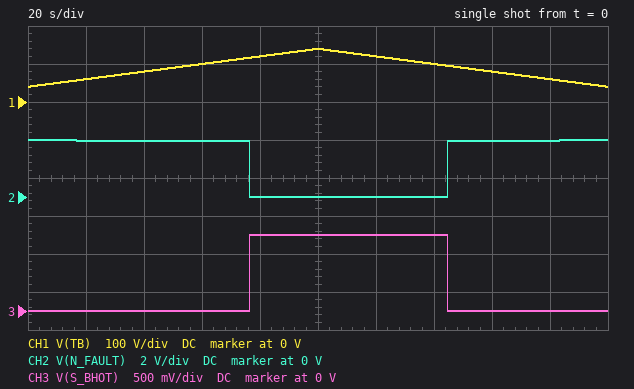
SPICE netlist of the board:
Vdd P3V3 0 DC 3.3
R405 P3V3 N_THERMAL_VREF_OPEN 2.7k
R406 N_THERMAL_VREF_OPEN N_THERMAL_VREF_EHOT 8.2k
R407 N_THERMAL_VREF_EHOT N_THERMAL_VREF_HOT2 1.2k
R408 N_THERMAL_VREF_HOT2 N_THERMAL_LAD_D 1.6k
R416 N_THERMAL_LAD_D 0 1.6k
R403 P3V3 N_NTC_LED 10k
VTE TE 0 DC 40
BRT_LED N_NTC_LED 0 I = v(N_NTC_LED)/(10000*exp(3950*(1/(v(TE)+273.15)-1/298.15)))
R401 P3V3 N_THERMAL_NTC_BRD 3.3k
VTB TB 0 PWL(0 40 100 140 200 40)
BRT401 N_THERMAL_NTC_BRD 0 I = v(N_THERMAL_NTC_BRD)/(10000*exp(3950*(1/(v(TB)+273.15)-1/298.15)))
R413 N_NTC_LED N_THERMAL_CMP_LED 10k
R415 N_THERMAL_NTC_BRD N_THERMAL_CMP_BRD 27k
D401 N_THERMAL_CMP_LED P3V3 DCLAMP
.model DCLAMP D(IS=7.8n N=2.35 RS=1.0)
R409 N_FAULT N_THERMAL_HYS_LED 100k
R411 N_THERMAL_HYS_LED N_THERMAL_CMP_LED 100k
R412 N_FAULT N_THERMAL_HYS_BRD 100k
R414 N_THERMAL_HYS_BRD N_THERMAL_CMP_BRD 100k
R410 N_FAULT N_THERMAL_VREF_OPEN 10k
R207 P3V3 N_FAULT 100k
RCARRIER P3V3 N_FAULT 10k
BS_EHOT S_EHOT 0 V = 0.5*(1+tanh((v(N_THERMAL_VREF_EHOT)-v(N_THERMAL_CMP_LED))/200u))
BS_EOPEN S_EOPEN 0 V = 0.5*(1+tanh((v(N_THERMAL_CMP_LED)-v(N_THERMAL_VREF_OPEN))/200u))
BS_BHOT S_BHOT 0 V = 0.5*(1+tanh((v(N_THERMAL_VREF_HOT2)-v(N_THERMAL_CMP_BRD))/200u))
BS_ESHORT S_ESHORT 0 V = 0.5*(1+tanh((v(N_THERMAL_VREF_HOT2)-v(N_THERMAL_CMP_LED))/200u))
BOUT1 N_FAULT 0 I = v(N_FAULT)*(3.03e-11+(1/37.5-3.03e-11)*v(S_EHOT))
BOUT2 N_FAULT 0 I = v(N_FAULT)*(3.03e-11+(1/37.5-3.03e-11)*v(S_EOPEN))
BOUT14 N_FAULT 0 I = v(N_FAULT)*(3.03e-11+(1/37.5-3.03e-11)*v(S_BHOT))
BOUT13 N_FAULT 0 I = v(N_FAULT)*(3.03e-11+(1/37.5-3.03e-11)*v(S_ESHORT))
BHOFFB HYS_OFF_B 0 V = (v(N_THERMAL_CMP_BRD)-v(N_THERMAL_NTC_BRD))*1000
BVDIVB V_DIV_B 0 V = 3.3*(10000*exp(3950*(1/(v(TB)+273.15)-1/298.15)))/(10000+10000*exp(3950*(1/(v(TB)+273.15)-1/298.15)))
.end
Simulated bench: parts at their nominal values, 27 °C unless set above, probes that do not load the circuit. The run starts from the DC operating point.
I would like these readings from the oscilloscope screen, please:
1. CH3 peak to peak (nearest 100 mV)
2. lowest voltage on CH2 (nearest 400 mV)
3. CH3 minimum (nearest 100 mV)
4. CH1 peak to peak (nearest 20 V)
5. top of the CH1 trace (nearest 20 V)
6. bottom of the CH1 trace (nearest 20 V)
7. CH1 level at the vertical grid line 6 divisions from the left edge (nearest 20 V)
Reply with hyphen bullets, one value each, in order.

- 1.0 V
- 0 V
- 0 V
- 100 V
- 140 V
- 40 V
- 120 V
